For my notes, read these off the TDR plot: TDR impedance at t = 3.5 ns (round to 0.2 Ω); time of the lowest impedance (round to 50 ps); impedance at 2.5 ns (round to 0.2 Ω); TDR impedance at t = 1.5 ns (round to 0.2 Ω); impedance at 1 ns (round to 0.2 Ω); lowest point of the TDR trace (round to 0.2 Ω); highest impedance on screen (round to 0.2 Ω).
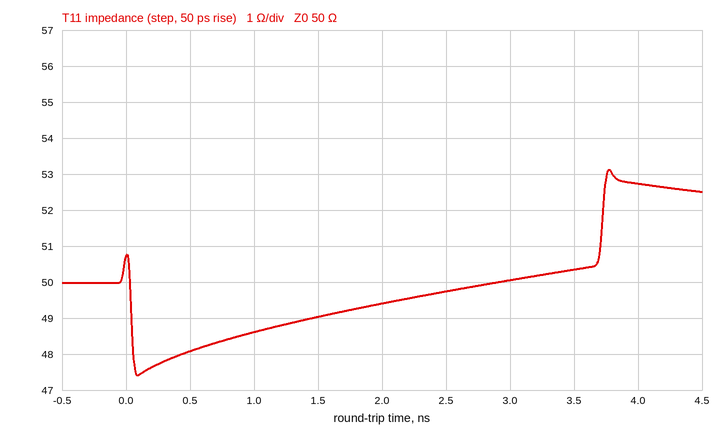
50.4 Ω
100 ps
49.8 Ω
49.0 Ω
48.6 Ω
47.4 Ω
53.2 Ω
